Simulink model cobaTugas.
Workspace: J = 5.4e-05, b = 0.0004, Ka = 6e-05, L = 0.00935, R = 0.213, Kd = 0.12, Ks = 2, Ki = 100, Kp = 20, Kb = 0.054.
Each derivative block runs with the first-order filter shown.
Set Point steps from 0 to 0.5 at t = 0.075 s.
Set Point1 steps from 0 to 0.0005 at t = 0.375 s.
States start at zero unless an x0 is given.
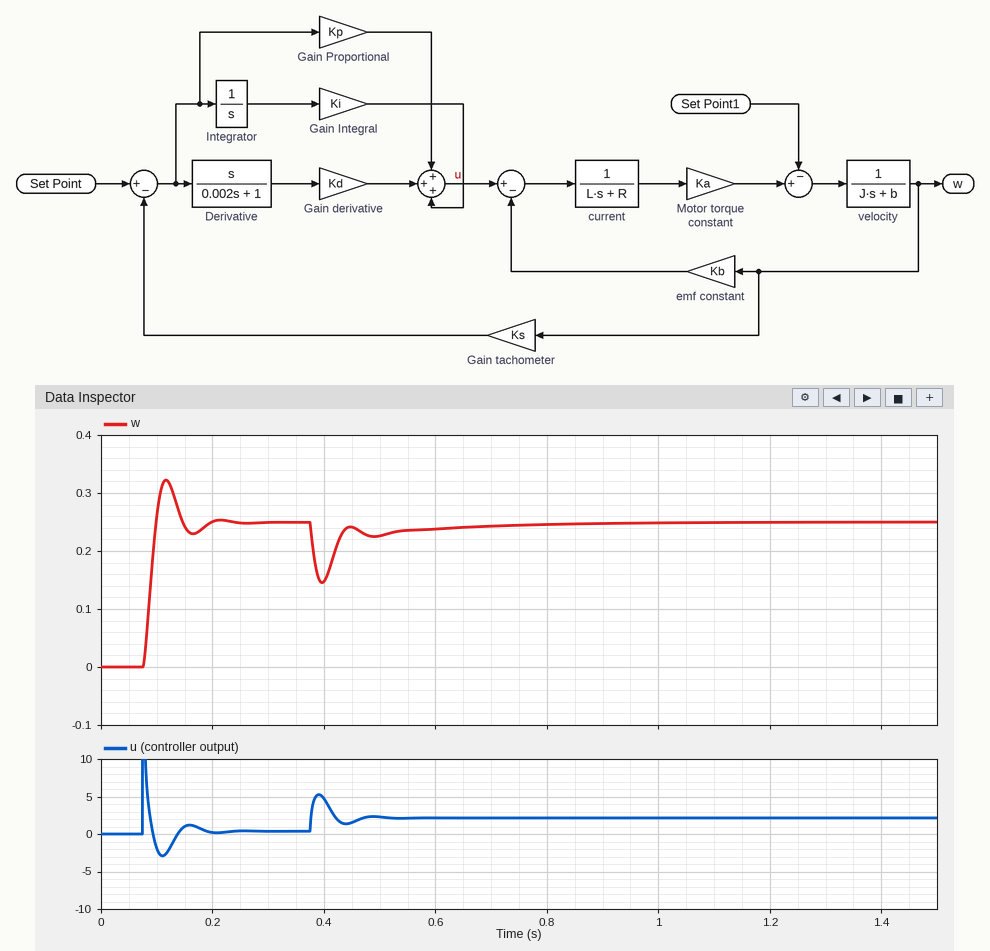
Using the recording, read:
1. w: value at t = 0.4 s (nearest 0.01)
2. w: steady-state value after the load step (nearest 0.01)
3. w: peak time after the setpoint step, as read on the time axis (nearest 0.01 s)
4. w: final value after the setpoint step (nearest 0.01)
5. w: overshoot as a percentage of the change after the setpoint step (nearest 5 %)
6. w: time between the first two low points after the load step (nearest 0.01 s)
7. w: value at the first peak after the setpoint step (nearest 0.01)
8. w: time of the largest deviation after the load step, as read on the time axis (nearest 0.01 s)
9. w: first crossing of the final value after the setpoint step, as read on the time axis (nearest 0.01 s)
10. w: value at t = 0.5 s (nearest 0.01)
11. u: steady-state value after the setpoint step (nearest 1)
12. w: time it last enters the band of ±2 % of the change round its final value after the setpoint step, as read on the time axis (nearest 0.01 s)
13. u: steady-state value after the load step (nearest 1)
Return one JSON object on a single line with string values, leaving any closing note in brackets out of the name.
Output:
{"w: value at t = 0.4 s": "0.15", "w: steady-state value after the load step": "0.25", "w: peak time after the setpoint step, as read on the time axis": "0.12 s", "w: final value after the setpoint step": "0.25", "w: overshoot as a percentage of the change after the setpoint step": "30 %", "w: time between the first two low points after the load step": "0.09 s", "w: value at the first peak after the setpoint step": "0.32", "w: time of the largest deviation after the load step, as read on the time axis": "0.40 s", "w: first crossing of the final value after the setpoint step, as read on the time axis": "0.10 s", "w: value at t = 0.5 s": "0.23", "u: steady-state value after the setpoint step": "0", "w: time it last enters the band of ±2 % of the change round its final value after the setpoint step, as read on the time axis": "0.19 s", "u: steady-state value after the load step": "2"}
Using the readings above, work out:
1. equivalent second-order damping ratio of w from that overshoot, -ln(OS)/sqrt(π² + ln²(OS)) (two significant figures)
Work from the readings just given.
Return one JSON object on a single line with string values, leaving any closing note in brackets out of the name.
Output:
{"equivalent second-order damping ratio of w from that overshoot, -ln(OS)/sqrt(π² + ln²(OS))": "0.36"}
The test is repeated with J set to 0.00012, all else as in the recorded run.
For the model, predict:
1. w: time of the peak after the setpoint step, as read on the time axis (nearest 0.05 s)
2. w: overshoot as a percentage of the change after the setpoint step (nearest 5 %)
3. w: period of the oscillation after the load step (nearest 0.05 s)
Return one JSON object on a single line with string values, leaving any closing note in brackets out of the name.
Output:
{"w: time of the peak after the setpoint step, as read on the time axis": "0.15 s", "w: overshoot as a percentage of the change after the setpoint step": "30 %", "w: period of the oscillation after the load step": "0.15 s"}
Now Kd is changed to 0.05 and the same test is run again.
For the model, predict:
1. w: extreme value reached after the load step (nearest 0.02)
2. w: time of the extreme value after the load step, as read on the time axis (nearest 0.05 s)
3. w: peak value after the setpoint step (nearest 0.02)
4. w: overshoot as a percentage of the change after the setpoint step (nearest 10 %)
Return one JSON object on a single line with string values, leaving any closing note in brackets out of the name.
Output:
{"w: extreme value reached after the load step": "0.14", "w: time of the extreme value after the load step, as read on the time axis": "0.40 s", "w: peak value after the setpoint step": "0.36", "w: overshoot as a percentage of the change after the setpoint step": "40 %"}
